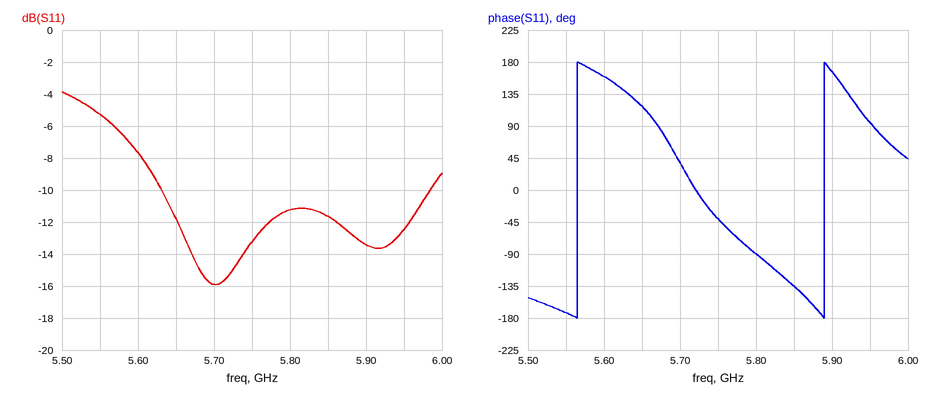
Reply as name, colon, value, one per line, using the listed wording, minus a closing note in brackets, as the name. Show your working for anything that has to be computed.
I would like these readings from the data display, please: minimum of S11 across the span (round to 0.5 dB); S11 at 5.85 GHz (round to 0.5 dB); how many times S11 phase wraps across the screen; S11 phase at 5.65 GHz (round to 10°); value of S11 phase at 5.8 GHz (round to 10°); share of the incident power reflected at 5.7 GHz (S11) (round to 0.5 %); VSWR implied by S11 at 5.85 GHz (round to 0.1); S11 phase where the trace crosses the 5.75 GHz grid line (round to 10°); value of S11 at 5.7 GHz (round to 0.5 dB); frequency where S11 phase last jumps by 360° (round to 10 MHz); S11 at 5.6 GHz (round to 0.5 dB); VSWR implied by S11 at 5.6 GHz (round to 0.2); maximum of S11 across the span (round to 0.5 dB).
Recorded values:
minimum of S11 across the span: -16.0 dB
S11 at 5.85 GHz: -11.5 dB
how many times S11 phase wraps across the screen: 2
S11 phase at 5.65 GHz: 120°
value of S11 phase at 5.8 GHz: -90°
share of the incident power reflected at 5.7 GHz (S11): 10^(-16/10) ≈ 2.5 %
VSWR implied by S11 at 5.85 GHz: |Γ| = 10^(-11.5/20) = 0.2661; VSWR = (1 + 0.2661)/(1 − 0.2661) ≈ 1.7
S11 phase where the trace crosses the 5.75 GHz grid line: -40°
value of S11 at 5.7 GHz: -16.0 dB
frequency where S11 phase last jumps by 360°: 5.89 GHz
S11 at 5.6 GHz: -7.5 dB
VSWR implied by S11 at 5.6 GHz: |Γ| = 10^(-7.5/20) = 0.4217; VSWR = (1 + 0.4217)/(1 − 0.4217) ≈ 2.46, so 2.4 to the nearest 0.2
maximum of S11 across the span: -4.0 dB
